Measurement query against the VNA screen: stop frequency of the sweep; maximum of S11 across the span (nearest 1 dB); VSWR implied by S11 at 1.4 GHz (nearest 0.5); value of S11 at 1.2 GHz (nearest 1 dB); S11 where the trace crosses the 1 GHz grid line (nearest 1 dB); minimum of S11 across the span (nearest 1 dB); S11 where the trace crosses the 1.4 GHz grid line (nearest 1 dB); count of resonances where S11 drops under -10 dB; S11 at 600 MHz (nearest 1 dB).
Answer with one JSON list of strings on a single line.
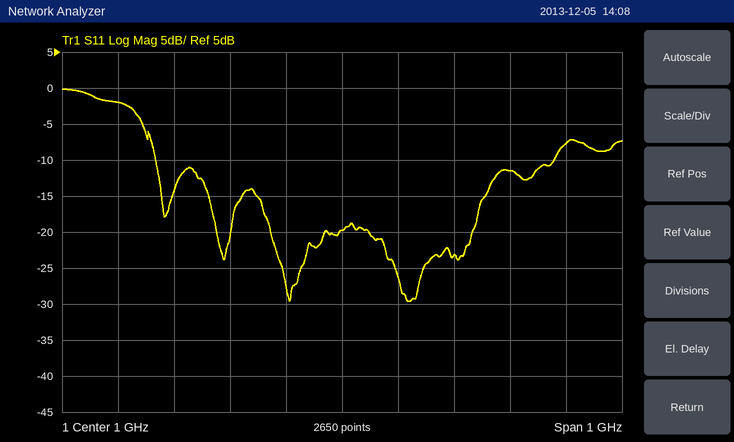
["1.5 GHz", "0 dB", "2.5", "-23 dB", "-20 dB", "-30 dB", "-8 dB", "4", "-2 dB"]
